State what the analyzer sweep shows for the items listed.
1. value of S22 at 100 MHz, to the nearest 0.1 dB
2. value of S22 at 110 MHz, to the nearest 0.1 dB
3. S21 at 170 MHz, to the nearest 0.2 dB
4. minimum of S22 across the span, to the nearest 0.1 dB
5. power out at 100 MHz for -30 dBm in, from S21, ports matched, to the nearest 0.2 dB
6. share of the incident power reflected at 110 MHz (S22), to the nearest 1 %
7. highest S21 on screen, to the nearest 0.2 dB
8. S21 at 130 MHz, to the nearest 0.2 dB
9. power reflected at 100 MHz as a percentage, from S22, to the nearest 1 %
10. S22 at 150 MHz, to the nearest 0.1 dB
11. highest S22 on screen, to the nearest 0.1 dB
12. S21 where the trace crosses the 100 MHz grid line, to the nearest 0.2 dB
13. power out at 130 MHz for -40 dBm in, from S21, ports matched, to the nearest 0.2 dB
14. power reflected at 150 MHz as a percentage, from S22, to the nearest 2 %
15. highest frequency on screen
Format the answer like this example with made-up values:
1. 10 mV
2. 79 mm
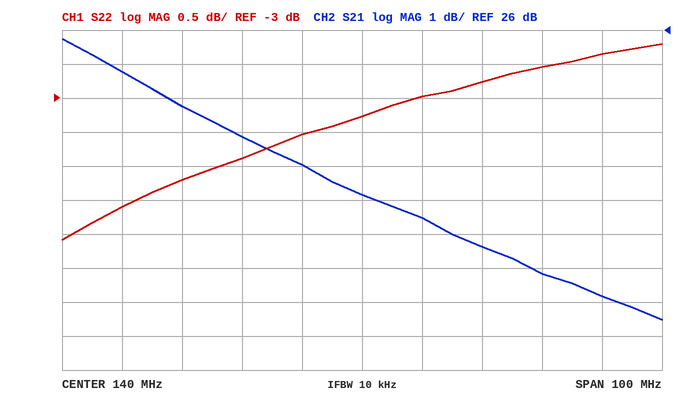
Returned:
1. -4.6 dB
2. -4.2 dB
3. 18.8 dB
4. -5.1 dB
5. -5.2 dBm
6. 38 %
7. 25.8 dB
8. 22.0 dB
9. 35 %
10. -3.0 dB
11. -2.2 dB
12. 24.8 dB
13. -18.0 dBm
14. 50 %
15. 190 MHz
